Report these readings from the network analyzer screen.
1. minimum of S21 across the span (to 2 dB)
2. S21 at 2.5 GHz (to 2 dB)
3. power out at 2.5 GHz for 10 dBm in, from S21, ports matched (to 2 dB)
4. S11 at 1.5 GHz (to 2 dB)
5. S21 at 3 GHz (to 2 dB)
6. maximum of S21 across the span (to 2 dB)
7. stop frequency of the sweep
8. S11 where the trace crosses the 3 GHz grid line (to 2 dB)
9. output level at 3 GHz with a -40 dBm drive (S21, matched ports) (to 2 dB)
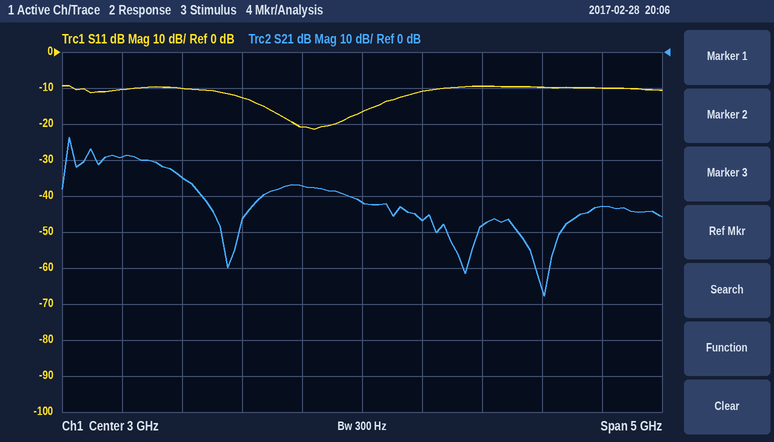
-68 dB
-38 dB
-28 dBm
-10 dB
-42 dB
-24 dB
5.5 GHz
-16 dB
-82 dBm
